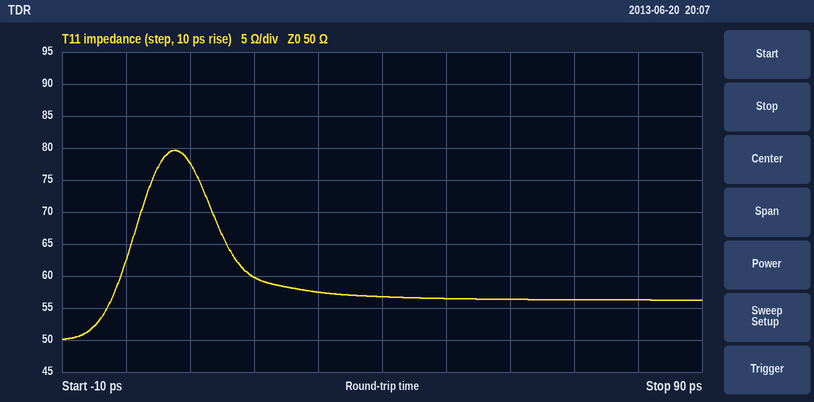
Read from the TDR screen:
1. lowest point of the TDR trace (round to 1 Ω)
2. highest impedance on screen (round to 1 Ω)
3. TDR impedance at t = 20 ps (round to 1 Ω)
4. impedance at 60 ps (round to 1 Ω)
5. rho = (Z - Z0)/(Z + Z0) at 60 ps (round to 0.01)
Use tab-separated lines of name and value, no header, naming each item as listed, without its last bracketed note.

lowest point of the TDR trace	50 Ω
highest impedance on screen	80 Ω
TDR impedance at t = 20 ps	60 Ω
impedance at 60 ps	56 Ω
rho = (Z - Z0)/(Z + Z0) at 60 ps	+0.06
